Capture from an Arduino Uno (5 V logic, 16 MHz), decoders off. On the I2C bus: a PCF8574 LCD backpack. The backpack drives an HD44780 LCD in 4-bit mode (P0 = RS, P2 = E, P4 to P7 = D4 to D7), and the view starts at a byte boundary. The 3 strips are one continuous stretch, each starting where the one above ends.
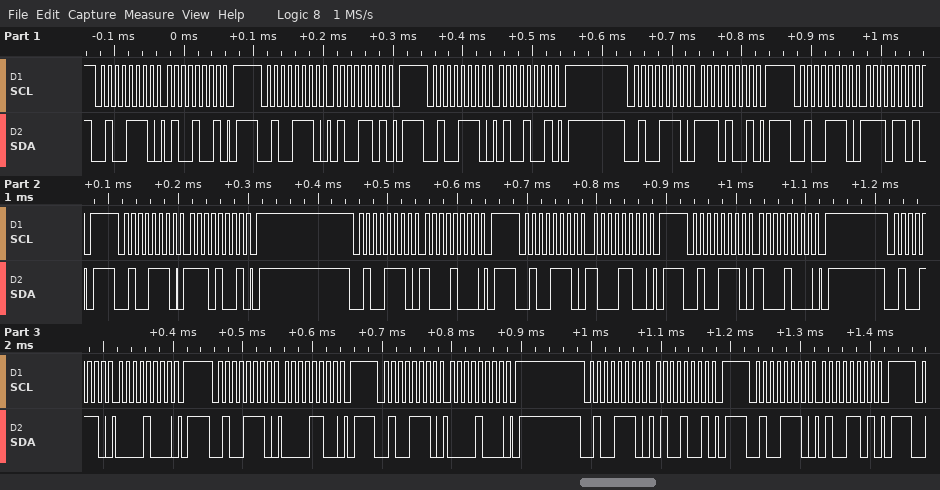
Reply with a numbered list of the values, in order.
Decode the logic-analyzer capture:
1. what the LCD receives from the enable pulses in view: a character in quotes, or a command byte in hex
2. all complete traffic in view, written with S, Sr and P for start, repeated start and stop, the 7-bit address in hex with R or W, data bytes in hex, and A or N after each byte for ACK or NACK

1. 'N' 0x80
2. S 27W A 49 A P S 27W A 4D A P S 27W A 49 A P S 27W A E9 A P S 27W A ED A P S 27W A E9 A P S 27W A 88 A P S 27W A 8C A P S 27W A 88 A P S 27W A 08 A P S 27W A 0C A P S 27W A 08 A P S 27W A 49 A P S 27W A 4D A P
